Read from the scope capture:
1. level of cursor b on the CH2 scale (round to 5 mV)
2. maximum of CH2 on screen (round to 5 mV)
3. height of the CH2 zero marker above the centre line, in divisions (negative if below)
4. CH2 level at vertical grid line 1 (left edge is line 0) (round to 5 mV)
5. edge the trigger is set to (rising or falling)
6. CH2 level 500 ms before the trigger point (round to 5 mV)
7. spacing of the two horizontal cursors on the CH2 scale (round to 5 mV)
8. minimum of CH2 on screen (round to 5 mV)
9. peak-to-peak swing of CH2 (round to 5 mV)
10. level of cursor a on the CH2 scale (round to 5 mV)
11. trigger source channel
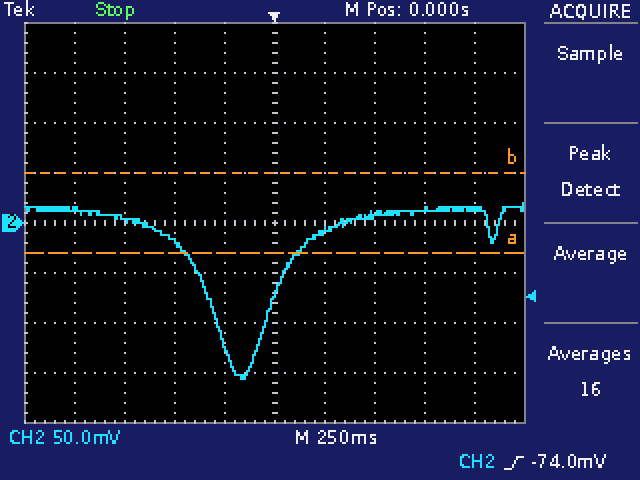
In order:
50 mV
20 mV
0.0 div
15 mV
rising
-20 mV
80 mV
-155 mV
175 mV
-30 mV
CH2
